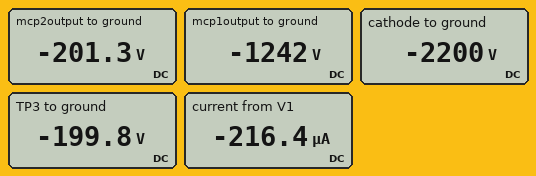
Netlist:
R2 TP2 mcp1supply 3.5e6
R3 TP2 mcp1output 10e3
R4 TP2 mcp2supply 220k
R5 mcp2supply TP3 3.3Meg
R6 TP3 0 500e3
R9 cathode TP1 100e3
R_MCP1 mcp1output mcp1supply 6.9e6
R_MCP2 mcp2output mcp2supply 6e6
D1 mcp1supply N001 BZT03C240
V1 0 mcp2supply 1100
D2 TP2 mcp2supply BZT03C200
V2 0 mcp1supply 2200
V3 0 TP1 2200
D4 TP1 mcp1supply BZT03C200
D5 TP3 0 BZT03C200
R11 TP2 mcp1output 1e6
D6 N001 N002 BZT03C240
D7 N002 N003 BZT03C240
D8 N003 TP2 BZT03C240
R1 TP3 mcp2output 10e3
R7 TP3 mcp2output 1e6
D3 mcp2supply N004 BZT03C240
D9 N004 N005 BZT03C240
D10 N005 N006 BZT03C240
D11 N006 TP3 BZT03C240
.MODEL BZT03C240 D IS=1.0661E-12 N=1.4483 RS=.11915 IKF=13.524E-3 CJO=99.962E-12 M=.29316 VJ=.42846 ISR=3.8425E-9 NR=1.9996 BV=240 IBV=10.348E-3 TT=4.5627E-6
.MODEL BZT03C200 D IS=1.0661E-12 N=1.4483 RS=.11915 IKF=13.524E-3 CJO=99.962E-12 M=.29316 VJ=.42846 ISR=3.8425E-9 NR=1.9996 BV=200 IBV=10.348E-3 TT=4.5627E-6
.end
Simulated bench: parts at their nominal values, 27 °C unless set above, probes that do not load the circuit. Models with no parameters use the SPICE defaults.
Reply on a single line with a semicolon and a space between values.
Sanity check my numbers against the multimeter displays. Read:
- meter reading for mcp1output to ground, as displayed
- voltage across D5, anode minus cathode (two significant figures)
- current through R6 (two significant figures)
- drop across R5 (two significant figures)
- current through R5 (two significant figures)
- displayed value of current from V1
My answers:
-1242 V; -200 V; 400 µA; 900 V; 270 µA; -216.4 µA
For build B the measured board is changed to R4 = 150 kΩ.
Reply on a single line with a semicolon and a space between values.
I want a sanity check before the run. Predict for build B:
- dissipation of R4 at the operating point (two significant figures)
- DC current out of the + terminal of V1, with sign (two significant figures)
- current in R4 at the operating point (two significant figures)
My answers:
130 mW; -510 µA; 940 µA
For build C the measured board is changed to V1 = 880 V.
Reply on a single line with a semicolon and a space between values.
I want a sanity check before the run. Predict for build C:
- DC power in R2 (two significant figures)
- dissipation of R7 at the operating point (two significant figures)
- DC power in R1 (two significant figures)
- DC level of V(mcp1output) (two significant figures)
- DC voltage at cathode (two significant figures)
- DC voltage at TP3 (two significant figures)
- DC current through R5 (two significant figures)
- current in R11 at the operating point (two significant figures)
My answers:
340 mW; 1.4 µW; 140 µW; -1.1 kV; -2.2 kV; -170 V; 220 µA; 1.6 µA
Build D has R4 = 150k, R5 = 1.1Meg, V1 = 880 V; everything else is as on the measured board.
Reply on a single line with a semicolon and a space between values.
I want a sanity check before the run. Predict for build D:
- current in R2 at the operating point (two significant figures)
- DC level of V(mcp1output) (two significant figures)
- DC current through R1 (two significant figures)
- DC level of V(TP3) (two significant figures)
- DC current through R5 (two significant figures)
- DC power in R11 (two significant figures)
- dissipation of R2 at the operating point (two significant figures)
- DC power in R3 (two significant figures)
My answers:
310 µA; -1.1 kV; 110 µA; -200 V; 620 µA; 2.4 µW; 340 mW; 240 µW
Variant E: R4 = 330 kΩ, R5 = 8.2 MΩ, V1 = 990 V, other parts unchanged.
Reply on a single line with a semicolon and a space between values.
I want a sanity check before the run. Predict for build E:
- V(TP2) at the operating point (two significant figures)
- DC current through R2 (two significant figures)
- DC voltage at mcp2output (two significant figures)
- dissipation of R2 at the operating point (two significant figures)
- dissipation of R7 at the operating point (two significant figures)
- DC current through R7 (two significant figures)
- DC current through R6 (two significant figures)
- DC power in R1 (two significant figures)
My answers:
-1.2 kV; 290 µA; -130 V; 290 mW; 2.0 µW; 1.4 µA; 250 µA; 200 µW
